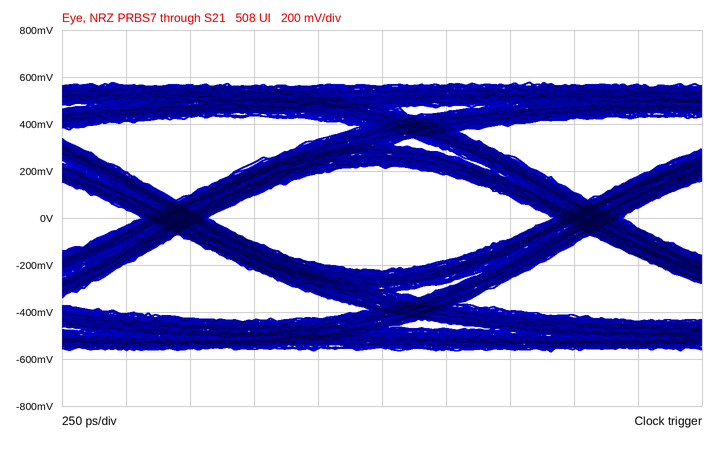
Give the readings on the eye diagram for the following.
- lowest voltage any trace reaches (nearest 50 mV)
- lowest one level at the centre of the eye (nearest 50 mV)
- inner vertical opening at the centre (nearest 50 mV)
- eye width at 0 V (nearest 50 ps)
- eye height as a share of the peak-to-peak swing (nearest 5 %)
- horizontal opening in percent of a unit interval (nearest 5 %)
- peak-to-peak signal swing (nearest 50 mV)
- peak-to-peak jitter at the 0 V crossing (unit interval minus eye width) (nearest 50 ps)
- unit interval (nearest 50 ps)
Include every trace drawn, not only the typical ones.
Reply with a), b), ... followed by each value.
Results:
a) -550 mV
b) 200 mV
c) 450 mV
d) 1.35 ns
e) 40 %
f) 85 %
g) 1.15 V
h) 250 ps
i) 1.60 ns
